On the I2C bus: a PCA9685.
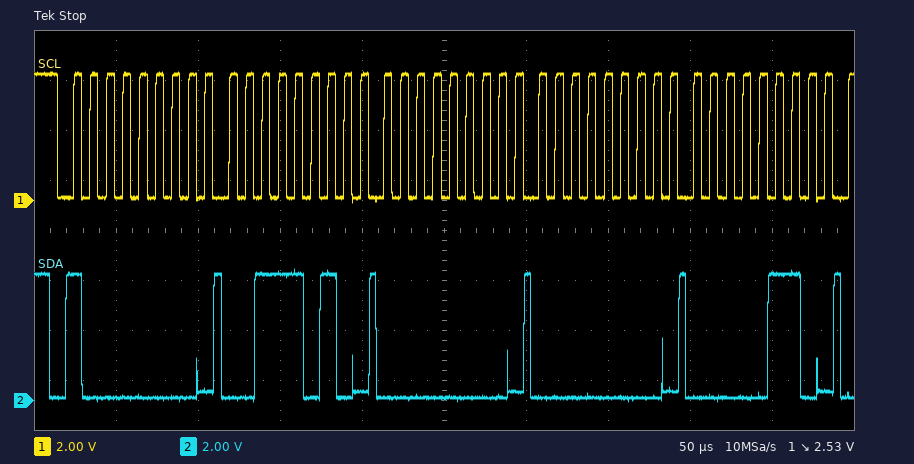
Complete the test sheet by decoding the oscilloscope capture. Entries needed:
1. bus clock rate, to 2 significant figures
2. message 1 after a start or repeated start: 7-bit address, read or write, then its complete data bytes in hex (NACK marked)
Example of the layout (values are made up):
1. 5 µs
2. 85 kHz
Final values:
1. 100 kHz
2. 0x40 write: 3A 00 00 06
